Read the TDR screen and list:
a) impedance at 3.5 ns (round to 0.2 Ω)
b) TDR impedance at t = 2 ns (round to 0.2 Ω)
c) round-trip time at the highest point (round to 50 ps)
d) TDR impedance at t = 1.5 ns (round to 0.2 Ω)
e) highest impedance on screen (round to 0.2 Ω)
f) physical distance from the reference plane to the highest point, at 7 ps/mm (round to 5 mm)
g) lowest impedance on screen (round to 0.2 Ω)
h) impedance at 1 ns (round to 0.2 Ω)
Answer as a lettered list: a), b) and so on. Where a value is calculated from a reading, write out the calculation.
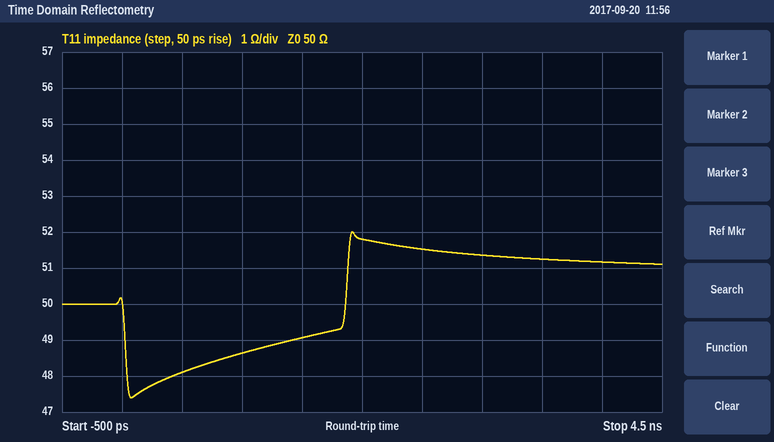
a) 51.2 Ω
b) 51.8 Ω
c) 1.90 ns
d) 49.0 Ω
e) 52.0 Ω
f) 1.90 ns / 2 / 7 ps/mm ≈ 136 mm, so 135 mm to the nearest 5 mm
g) 47.4 Ω
h) 48.6 Ω
